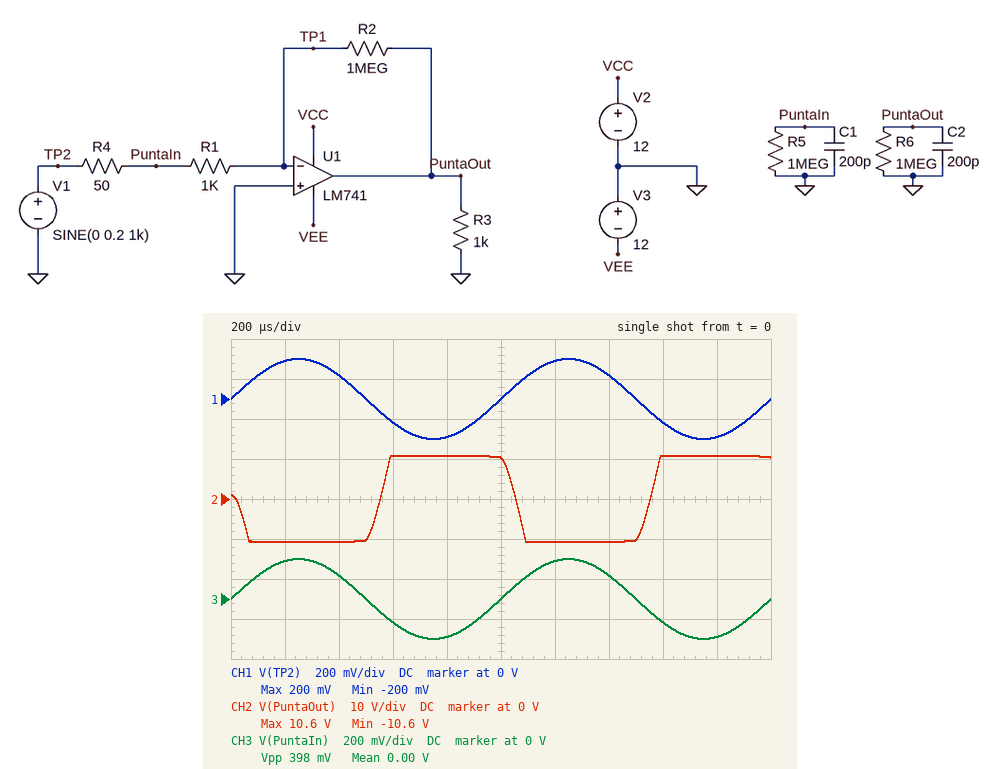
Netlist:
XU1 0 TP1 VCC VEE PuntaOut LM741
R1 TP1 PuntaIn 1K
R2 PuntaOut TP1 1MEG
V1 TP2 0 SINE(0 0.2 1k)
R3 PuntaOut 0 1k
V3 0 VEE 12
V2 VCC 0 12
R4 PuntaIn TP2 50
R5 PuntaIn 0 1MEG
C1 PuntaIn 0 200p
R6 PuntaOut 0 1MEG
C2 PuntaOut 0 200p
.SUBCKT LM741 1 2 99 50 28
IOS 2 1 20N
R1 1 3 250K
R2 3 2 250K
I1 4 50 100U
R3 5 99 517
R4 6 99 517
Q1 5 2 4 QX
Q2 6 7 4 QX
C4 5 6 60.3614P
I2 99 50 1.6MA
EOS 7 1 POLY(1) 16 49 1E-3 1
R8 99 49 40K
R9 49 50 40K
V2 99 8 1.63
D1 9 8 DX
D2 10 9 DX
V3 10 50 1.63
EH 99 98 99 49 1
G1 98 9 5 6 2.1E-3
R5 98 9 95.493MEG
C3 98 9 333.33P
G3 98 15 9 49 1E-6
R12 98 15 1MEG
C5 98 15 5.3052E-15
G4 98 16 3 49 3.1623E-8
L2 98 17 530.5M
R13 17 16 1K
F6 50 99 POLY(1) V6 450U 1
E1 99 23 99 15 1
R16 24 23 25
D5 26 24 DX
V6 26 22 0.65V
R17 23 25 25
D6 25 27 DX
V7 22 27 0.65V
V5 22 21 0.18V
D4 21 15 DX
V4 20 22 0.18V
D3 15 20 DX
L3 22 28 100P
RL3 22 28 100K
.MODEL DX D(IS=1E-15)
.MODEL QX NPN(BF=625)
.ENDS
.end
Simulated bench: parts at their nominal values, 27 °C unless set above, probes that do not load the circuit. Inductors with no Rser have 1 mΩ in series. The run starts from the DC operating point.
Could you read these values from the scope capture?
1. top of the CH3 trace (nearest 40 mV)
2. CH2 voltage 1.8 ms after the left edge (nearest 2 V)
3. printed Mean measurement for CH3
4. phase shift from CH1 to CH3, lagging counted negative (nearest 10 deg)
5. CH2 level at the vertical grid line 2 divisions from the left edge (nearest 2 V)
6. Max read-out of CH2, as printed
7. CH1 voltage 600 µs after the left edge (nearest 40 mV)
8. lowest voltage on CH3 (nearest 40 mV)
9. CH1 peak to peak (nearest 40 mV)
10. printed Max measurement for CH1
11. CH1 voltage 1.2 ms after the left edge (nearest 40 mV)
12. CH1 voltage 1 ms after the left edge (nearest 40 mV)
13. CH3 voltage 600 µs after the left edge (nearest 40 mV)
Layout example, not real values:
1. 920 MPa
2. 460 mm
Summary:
1. 200 mV
2. 10 V
3. 0.00 V
4. 0 deg
5. -10 V
6. 10.6 V
7. -120 mV
8. -200 mV
9. 400 mV
10. 200 mV
11. 200 mV
12. 0 V
13. -120 mV
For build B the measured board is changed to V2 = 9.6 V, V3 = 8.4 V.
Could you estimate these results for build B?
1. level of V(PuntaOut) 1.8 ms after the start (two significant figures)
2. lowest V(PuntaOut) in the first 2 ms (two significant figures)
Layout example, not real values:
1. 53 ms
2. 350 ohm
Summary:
1. 8.3 V
2. -7.1 V
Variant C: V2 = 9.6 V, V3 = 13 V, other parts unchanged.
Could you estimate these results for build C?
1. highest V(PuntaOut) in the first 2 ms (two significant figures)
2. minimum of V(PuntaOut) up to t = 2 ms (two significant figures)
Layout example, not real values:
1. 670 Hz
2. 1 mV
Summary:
1. 8.3 V
2. -12 V
